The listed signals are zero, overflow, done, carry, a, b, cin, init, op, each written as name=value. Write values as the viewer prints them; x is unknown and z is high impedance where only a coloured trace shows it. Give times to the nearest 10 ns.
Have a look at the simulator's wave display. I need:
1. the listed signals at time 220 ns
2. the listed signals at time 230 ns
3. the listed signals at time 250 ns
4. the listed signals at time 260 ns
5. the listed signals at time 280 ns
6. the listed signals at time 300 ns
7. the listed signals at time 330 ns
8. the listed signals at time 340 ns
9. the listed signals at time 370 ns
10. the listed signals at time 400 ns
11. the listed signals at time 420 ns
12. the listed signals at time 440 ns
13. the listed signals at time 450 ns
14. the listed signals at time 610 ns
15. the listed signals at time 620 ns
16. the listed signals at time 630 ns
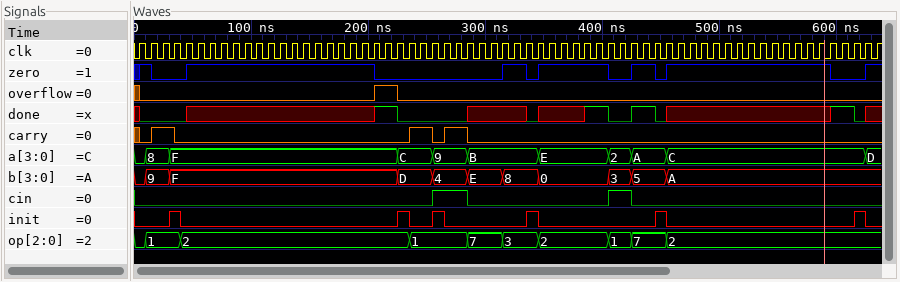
zero=0, overflow=1, done=1, carry=0, a=F, b=F, cin=0, init=0, op=2
zero=0, overflow=0, done=0, carry=0, a=C, b=D, cin=0, init=1, op=2
zero=0, overflow=0, done=0, carry=1, a=C, b=D, cin=0, init=0, op=1
zero=0, overflow=0, done=0, carry=0, a=9, b=4, cin=1, init=1, op=1
zero=0, overflow=0, done=0, carry=1, a=9, b=4, cin=1, init=0, op=1
zero=0, overflow=0, done=x, carry=0, a=B, b=E, cin=0, init=0, op=7
zero=1, overflow=0, done=x, carry=0, a=B, b=8, cin=0, init=0, op=3
zero=0, overflow=0, done=0, carry=0, a=B, b=8, cin=0, init=1, op=3
zero=1, overflow=0, done=x, carry=0, a=E, b=0, cin=0, init=0, op=2
zero=1, overflow=0, done=1, carry=0, a=E, b=0, cin=0, init=0, op=2
zero=0, overflow=0, done=0, carry=0, a=2, b=3, cin=1, init=0, op=1
zero=1, overflow=0, done=1, carry=0, a=A, b=5, cin=0, init=0, op=7
zero=0, overflow=0, done=0, carry=0, a=A, b=5, cin=0, init=1, op=7
zero=0, overflow=0, done=1, carry=0, a=C, b=A, cin=0, init=0, op=2
zero=0, overflow=0, done=0, carry=0, a=C, b=A, cin=0, init=1, op=2
zero=1, overflow=0, done=x, carry=0, a=D, b=A, cin=0, init=0, op=2
